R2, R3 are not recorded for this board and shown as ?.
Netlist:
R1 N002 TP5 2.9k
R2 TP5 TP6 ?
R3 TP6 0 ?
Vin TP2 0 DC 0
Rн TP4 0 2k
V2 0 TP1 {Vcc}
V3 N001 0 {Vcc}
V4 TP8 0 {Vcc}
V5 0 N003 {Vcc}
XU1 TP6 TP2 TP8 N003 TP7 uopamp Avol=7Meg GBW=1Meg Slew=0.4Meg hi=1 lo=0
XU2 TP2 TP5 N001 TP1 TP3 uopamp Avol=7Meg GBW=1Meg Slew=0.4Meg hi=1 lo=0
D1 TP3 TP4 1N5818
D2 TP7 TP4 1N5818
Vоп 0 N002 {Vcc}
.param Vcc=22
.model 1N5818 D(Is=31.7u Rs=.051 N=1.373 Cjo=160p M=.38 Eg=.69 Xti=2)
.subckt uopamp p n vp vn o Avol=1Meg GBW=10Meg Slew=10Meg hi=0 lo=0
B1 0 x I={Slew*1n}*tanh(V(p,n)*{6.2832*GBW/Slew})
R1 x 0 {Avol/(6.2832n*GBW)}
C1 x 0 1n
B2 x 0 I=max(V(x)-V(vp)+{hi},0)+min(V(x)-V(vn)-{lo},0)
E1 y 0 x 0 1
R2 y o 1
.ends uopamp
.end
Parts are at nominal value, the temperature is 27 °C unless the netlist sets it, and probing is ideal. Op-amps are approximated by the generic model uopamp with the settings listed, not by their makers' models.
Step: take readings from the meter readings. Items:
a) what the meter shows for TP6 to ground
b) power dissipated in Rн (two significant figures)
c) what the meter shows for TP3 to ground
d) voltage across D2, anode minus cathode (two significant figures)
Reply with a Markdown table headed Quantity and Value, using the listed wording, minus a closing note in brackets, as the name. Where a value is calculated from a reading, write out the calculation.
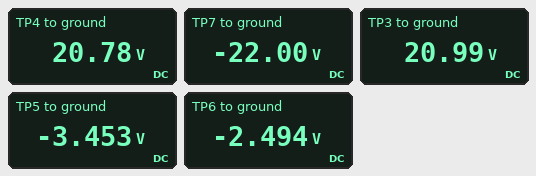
| Quantity | Value |
|---|---|
| what the meter shows for TP6 to ground | -2.494 V |
| power dissipated in Rн | (20.78 V)^2 / 2 kΩ = 220 mW |
| what the meter shows for TP3 to ground | 20.99 V |
| voltage across D2, anode minus cathode | -22 V - 20.78 V = -43 V |
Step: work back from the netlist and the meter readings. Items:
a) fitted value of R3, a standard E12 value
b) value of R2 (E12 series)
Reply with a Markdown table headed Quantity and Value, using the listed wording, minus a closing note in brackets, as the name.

| Quantity | Value |
|---|---|
| fitted value of R3, a standard E12 value | 390 Ω |
| value of R2 | 150 Ω |
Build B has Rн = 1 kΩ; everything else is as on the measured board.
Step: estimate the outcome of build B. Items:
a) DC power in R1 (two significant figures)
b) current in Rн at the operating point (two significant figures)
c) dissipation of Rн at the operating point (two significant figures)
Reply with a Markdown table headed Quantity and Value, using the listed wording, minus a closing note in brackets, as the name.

| Quantity | Value |
|---|---|
| DC power in R1 | 120 mW |
| current in Rн at the operating point | 21 mA |
| dissipation of Rн at the operating point | 430 mW |
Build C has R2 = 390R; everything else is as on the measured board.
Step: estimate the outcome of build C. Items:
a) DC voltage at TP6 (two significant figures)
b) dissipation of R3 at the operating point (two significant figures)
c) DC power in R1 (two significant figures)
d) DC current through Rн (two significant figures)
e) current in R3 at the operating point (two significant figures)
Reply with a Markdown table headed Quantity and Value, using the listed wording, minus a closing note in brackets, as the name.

| Quantity | Value |
|---|---|
| DC voltage at TP6 | -2.3 V |
| dissipation of R3 at the operating point | 14 mW |
| DC power in R1 | 100 mW |
| DC current through Rн | 10 mA |
| current in R3 at the operating point | 6.0 mA |
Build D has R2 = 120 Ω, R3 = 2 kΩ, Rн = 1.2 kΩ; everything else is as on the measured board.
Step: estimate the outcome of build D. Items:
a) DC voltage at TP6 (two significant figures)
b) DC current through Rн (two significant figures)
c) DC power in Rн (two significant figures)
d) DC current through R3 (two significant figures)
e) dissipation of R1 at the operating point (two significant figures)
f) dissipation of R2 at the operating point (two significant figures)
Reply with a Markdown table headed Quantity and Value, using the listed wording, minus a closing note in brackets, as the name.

| Quantity | Value |
|---|---|
| DC voltage at TP6 | -8.8 V |
| DC current through Rн | 17 mA |
| DC power in Rн | 360 mW |
| DC current through R3 | 4.4 mA |
| dissipation of R1 at the operating point | 56 mW |
| dissipation of R2 at the operating point | 2.3 mW |
